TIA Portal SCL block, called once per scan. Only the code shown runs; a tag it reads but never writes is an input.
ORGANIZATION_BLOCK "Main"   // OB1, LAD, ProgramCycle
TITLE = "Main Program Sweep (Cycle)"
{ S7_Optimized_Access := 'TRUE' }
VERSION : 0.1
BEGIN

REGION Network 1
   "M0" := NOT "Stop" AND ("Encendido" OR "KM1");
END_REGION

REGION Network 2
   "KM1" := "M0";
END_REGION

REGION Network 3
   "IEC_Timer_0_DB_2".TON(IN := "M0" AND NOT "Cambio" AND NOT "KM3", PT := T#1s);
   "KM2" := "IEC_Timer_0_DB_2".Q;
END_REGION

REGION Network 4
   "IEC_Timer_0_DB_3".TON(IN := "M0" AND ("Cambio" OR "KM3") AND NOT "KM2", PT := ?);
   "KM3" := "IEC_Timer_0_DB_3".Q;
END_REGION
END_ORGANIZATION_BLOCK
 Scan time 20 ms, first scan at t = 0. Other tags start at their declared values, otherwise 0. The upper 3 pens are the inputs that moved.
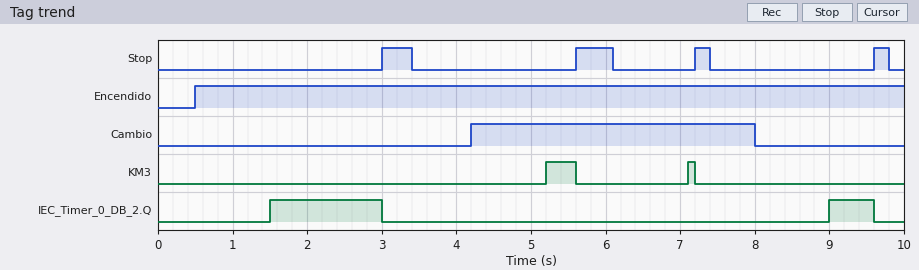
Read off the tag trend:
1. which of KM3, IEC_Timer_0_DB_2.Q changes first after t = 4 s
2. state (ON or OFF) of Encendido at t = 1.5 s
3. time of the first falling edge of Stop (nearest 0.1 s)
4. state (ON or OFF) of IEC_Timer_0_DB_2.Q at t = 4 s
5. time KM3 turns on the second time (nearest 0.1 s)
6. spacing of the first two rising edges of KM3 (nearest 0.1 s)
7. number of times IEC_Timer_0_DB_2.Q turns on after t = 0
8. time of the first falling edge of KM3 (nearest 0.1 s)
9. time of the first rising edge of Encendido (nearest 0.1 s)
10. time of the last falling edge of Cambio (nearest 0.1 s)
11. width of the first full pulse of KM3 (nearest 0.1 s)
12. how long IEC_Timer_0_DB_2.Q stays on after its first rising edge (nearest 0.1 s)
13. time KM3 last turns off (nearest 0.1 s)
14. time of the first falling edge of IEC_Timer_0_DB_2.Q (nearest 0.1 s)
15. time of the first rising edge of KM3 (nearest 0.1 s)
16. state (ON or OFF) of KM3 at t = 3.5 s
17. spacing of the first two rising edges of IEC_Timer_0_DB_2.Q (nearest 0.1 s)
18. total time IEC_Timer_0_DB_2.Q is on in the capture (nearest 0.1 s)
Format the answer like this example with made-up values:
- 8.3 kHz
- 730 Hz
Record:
- KM3
- ON
- 3.4 s
- OFF
- 7.1 s
- 1.9 s
- 2
- 5.6 s
- 0.5 s
- 8.0 s
- 0.4 s
- 1.5 s
- 7.2 s
- 3.0 s
- 5.2 s
- OFF
- 7.5 s
- 2.1 s
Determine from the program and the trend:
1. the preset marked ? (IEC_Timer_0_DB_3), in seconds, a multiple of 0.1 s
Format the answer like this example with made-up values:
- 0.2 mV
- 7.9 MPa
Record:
- 1.0 s
